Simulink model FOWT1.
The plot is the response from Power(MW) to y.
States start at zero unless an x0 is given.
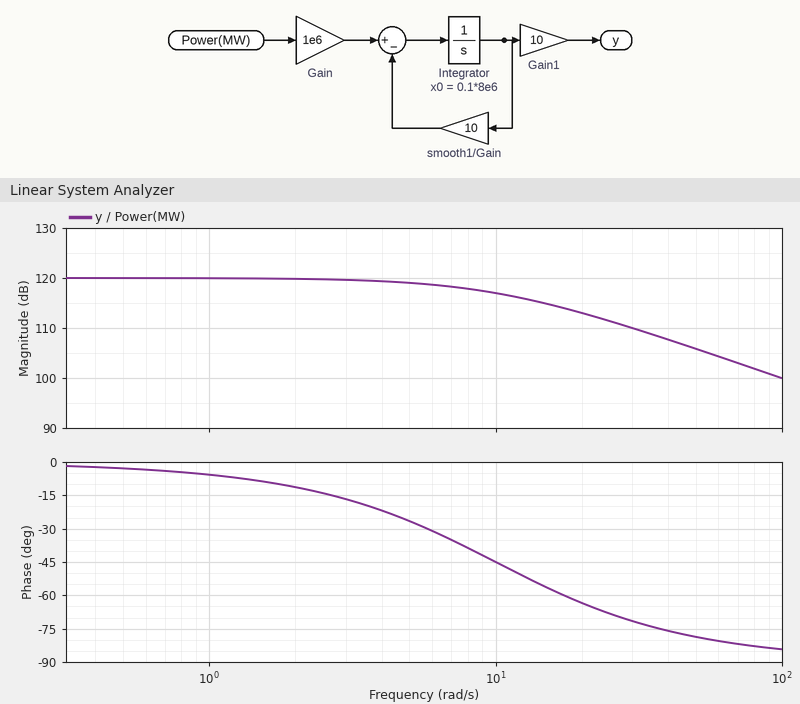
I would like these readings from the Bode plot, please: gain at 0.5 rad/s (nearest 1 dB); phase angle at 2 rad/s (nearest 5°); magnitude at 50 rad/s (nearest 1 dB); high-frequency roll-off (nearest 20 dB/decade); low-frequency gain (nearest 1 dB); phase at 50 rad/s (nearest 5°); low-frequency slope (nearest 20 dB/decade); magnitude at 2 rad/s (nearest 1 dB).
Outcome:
120 dB
-10°
106 dB
-20 dB/decade
120 dB
-80°
0 dB/decade
120 dB
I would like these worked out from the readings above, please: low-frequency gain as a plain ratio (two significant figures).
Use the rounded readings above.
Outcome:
1000000
